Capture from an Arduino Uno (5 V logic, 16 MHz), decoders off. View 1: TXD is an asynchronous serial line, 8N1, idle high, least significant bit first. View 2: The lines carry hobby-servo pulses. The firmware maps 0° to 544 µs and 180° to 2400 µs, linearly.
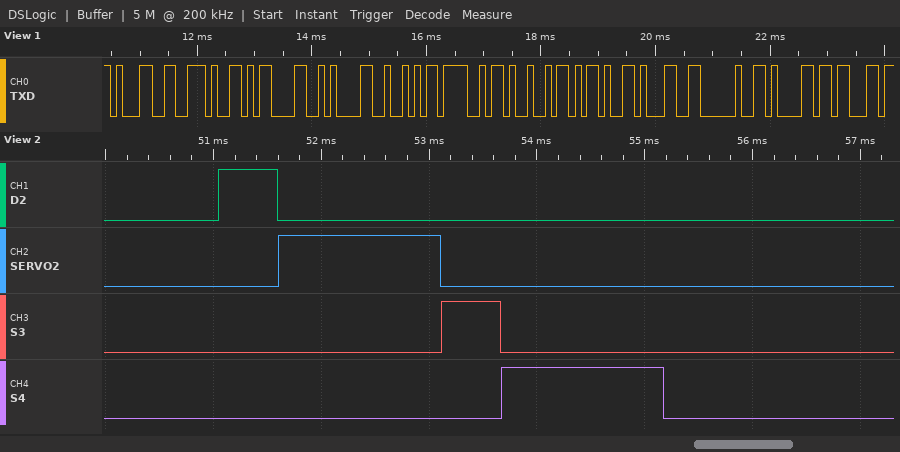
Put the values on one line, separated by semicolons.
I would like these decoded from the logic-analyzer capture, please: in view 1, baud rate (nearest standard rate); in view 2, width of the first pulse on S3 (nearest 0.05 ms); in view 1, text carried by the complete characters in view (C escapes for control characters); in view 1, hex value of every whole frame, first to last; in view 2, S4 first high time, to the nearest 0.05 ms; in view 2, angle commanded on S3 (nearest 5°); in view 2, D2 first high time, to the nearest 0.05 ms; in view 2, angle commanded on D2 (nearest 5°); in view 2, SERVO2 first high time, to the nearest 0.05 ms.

9600 baud; 0.55 ms; "1.\r\nROI-1 ac"; 31 2E 0D 0A 52 4F 49 2D 31 20 61 63; 1.50 ms; 0°; 0.55 ms; 0°; 1.50 ms
